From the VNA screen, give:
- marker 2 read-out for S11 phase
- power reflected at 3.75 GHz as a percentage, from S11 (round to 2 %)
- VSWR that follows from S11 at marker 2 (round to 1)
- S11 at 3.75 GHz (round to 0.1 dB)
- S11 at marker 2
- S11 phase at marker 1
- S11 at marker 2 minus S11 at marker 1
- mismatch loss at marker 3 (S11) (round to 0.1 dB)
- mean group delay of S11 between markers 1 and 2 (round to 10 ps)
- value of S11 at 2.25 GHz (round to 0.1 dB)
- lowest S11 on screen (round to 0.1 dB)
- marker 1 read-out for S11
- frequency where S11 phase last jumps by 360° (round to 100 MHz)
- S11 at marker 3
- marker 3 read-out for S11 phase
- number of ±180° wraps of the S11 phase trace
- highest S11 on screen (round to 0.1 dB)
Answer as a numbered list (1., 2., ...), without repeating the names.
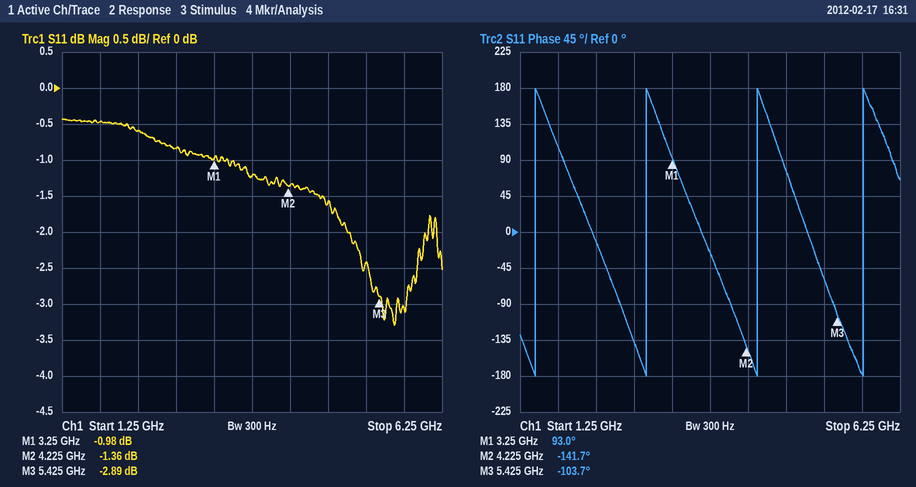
1. -141.7°
2. 76 %
3. 13
4. -1.2 dB
5. -1.36 dB
6. 93.0°
7. -0.38 dB
8. 3.1 dB
9. 670 ps
10. -0.6 dB
11. -3.3 dB
12. -0.98 dB
13. 5.8 GHz
14. -2.89 dB
15. -103.7°
16. 4
17. -0.4 dB
